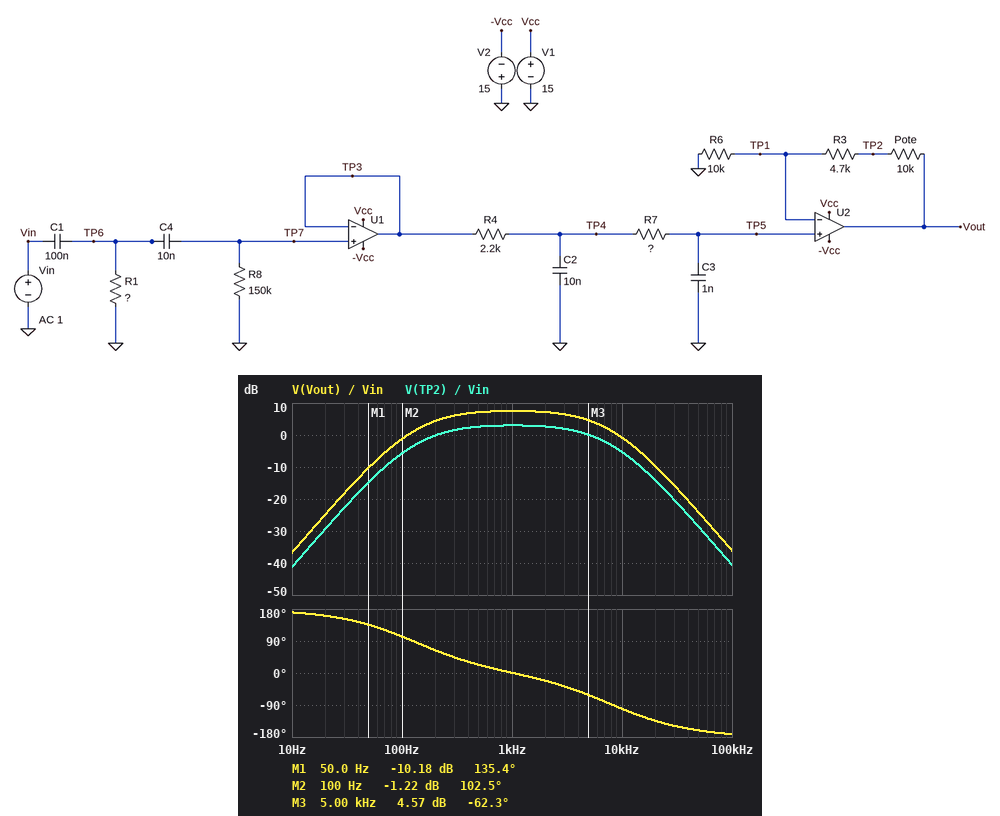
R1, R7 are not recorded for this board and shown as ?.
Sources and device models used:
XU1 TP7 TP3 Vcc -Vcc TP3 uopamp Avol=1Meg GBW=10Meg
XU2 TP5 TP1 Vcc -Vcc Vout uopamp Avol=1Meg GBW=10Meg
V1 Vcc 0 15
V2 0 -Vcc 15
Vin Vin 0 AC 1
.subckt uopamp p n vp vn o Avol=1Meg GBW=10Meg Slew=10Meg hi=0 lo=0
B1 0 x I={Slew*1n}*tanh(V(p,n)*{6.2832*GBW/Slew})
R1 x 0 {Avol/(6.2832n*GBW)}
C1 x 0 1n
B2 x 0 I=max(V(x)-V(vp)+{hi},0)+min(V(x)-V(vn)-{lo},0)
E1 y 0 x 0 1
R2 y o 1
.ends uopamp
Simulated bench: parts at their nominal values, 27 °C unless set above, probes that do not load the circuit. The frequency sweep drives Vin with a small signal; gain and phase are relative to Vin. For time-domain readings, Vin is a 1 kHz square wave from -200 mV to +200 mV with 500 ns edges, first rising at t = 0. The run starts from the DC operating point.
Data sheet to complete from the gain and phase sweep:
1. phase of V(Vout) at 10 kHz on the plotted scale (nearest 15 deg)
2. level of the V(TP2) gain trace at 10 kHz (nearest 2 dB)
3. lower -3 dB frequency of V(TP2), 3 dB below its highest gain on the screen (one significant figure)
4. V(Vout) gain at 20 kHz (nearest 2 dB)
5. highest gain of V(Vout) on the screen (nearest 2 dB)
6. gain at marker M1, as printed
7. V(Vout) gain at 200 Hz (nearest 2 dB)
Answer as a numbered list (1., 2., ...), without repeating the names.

1. -105 deg
2. -6 dB
3. 200 Hz
4. -10 dB
5. 8 dB
6. -10.18 dB
7. 4 dB
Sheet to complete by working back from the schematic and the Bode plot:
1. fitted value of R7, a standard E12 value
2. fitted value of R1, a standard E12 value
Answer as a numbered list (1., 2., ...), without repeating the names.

1. 18 kΩ
2. 10 kΩ
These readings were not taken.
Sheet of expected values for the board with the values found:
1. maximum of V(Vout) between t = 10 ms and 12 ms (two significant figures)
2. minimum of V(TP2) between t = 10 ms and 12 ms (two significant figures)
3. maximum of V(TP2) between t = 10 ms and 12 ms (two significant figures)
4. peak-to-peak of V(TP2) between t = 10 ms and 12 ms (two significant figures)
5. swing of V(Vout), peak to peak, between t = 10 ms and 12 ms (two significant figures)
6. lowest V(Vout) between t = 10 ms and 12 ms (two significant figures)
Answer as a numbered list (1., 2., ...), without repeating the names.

1. 590 mV
2. -350 mV
3. 350 mV
4. 700 mV
5. 1.2 V
6. -590 mV
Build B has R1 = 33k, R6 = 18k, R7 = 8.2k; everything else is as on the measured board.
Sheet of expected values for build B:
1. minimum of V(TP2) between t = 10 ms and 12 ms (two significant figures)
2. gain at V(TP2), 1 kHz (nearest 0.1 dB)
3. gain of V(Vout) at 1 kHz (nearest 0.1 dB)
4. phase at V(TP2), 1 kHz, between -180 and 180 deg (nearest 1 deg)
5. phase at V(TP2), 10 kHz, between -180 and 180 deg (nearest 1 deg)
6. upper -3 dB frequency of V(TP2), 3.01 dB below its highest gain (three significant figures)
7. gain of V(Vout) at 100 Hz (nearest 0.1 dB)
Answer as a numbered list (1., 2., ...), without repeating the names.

1. -290 mV
2. 1.8 dB
3. 5.0 dB
4. -2 deg
5. -81 deg
6. 6.11 kHz
7. 0.5 dB
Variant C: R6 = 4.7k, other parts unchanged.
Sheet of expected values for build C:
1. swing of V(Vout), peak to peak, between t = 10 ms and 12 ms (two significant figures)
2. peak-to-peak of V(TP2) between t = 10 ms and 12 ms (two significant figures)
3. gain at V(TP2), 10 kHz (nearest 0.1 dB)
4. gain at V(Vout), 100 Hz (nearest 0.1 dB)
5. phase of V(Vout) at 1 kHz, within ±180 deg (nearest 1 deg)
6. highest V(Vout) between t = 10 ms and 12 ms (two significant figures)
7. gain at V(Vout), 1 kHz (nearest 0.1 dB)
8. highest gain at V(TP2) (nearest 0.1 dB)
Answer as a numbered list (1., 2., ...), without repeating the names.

1. 2.0 V
2. 950 mV
3. -2.6 dB
4. 3.2 dB
5. 1 deg
6. 980 mV
7. 12.0 dB
8. 5.7 dB
